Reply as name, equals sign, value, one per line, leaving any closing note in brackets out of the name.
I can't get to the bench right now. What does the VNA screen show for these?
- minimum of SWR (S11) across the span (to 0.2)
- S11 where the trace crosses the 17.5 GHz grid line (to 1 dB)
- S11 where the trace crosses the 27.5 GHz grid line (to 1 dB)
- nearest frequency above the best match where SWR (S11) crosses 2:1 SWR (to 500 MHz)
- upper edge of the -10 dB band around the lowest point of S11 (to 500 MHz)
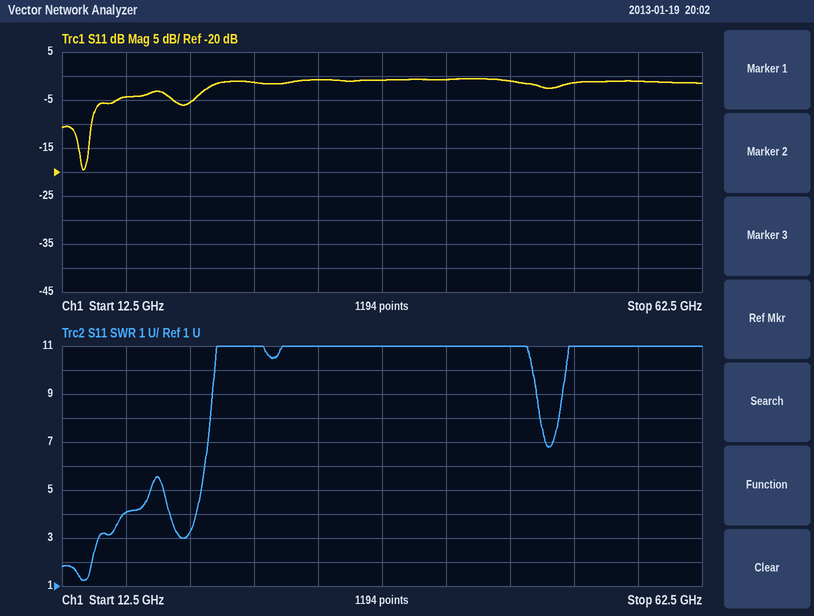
minimum of SWR (S11) across the span = 1.2
S11 where the trace crosses the 17.5 GHz grid line = -4 dB
S11 where the trace crosses the 27.5 GHz grid line = -1 dB
nearest frequency above the best match where SWR (S11) crosses 2:1 SWR = 15.0 GHz
upper edge of the -10 dB band around the lowest point of S11 = 15.0 GHz
